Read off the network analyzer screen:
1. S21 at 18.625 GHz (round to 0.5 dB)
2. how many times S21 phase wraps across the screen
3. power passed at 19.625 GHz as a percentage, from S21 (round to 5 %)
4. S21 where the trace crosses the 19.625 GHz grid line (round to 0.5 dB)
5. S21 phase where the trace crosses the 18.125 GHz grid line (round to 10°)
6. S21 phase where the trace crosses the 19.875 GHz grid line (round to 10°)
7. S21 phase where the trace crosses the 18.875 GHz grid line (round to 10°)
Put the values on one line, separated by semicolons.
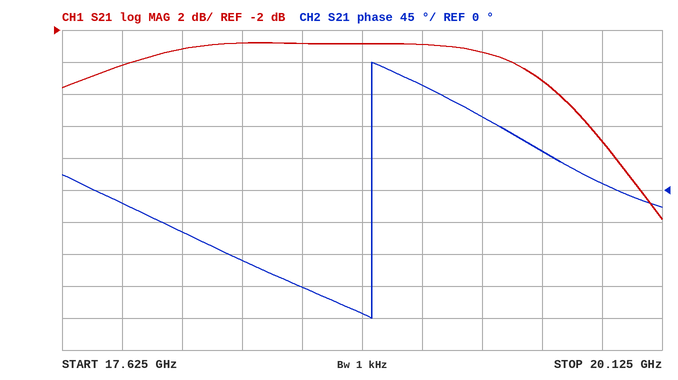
-3.0 dB; 1; 30 %; -5.0 dB; -60°; 10°; -170°
